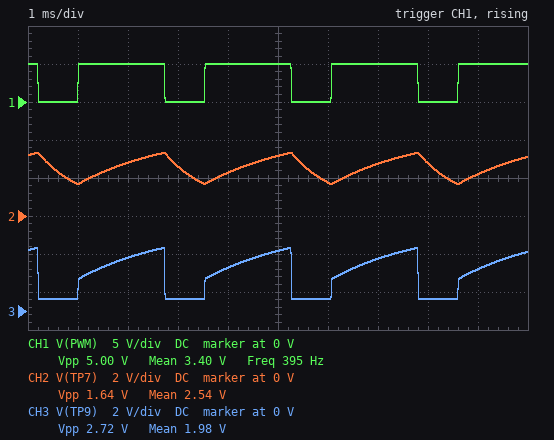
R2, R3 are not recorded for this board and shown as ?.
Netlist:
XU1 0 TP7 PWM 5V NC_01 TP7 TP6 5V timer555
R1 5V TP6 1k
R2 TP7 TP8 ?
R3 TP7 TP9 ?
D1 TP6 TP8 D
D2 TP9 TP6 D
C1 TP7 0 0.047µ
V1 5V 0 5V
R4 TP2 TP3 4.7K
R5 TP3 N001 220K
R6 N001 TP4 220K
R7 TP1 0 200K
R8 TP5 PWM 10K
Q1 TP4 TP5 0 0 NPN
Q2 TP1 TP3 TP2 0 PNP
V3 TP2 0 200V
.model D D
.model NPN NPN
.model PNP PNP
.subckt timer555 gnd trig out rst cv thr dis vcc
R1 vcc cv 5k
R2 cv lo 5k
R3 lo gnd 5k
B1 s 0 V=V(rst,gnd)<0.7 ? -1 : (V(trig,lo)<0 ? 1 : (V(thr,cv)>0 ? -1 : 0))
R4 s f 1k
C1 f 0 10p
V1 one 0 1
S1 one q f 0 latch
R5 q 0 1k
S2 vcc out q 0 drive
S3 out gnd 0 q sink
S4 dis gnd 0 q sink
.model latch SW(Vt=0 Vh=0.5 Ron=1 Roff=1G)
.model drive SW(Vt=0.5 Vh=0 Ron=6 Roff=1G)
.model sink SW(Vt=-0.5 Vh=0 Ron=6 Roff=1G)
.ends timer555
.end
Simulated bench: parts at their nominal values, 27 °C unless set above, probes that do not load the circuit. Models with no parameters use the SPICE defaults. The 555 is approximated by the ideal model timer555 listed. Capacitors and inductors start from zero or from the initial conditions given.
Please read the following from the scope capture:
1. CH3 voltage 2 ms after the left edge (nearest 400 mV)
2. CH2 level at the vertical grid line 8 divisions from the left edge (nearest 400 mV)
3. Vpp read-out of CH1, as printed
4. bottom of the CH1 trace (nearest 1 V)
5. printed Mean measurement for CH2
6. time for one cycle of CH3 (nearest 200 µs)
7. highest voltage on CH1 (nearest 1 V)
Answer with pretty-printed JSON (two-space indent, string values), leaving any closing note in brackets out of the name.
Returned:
{
  "CH3 voltage 2 ms after the left edge": "2.8 V",
  "CH2 level at the vertical grid line 8 divisions from the left edge": "2.8 V",
  "Vpp read-out of CH1, as printed": "5.00 V",
  "bottom of the CH1 trace": "0 V",
  "printed Mean measurement for CH2": "2.54 V",
  "time for one cycle of CH3": "2.6 ms",
  "highest voltage on CH1": "5 V"
}
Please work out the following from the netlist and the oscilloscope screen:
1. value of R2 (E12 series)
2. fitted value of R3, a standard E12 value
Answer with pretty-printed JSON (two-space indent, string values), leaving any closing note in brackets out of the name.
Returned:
{
  "value of R2": "39 kΩ",
  "fitted value of R3, a standard E12 value": "18 kΩ"
}
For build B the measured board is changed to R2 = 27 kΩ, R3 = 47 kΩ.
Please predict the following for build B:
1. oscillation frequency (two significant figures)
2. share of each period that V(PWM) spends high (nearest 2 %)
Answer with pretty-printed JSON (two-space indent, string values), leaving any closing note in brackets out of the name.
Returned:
{
  "oscillation frequency": "300 Hz",
  "share of each period that V(PWM) spends high": "38 %"
}
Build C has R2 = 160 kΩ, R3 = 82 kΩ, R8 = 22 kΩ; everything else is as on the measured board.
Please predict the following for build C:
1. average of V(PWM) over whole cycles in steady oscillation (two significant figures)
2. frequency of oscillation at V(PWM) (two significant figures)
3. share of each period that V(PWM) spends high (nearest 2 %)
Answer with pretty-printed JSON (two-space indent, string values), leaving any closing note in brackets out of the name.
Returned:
{
  "average of V(PWM) over whole cycles in steady oscillation": "3.3 V",
  "frequency of oscillation at V(PWM)": "96 Hz",
  "share of each period that V(PWM) spends high": "66 %"
}
